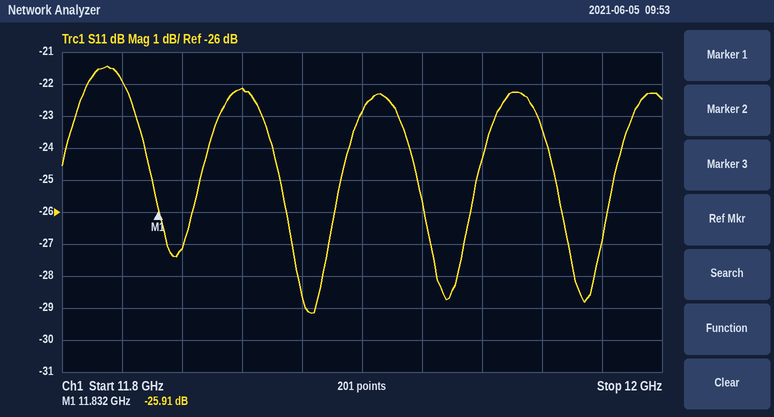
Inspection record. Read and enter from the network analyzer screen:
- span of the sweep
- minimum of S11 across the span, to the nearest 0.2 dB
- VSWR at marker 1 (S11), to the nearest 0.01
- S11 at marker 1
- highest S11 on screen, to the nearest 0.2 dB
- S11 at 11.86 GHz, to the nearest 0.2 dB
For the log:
200 MHz
-29.2 dB
1.11
-25.91 dB
-21.4 dB
-22.2 dB
